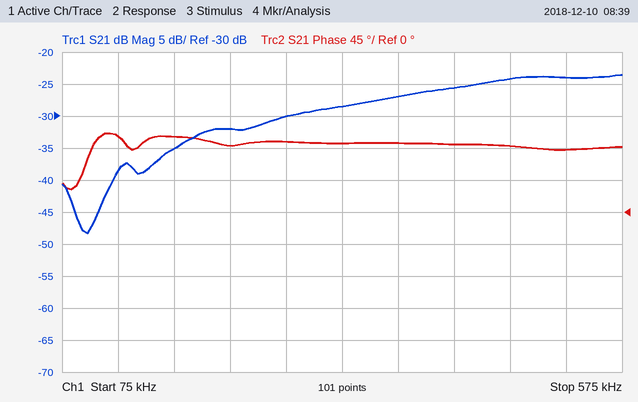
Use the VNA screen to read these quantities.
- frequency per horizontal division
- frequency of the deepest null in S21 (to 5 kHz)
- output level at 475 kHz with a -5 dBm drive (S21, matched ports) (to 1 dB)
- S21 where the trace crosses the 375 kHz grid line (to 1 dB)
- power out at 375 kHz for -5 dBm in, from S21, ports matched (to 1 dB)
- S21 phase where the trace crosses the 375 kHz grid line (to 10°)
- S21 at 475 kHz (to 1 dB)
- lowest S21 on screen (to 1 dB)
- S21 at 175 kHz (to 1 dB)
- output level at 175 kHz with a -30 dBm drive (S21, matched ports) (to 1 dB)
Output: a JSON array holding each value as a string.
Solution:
["50 kHz", "100 kHz", "-29 dBm", "-27 dB", "-32 dBm", "100°", "-24 dB", "-48 dB", "-35 dB", "-65 dBm"]
